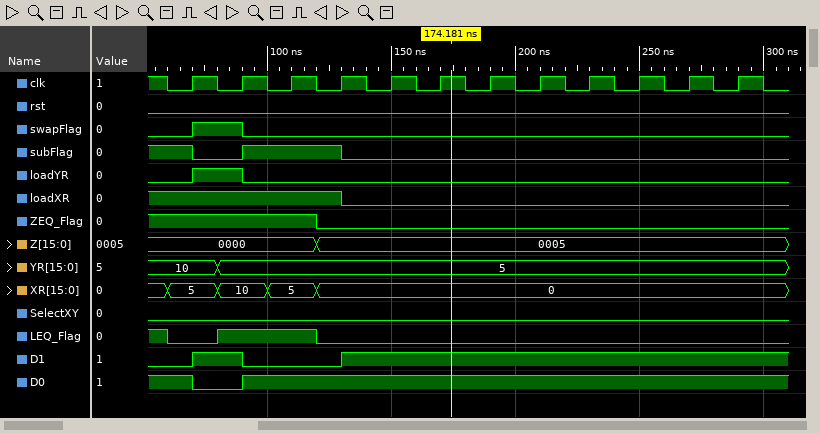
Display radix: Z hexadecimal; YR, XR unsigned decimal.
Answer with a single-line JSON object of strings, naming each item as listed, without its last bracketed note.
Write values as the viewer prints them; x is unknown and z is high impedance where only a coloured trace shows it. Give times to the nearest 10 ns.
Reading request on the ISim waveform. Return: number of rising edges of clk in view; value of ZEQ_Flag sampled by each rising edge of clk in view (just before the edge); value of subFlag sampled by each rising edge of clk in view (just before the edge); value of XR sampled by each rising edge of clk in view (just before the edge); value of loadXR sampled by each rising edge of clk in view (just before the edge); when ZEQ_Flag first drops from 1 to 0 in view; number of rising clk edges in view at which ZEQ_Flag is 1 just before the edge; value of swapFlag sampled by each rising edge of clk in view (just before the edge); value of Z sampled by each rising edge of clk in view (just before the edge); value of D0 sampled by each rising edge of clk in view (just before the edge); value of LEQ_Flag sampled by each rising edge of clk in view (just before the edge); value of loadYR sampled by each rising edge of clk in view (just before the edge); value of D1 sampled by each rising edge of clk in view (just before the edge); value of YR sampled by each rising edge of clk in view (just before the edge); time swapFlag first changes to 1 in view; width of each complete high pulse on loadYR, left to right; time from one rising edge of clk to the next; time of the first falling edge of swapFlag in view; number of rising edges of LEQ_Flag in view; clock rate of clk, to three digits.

{"number of rising edges of clk in view": "12", "value of ZEQ_Flag sampled by each rising edge of clk in view": "1 1 1 0 0 0 0 0 0 0 0 0", "value of subFlag sampled by each rising edge of clk in view": "1 0 1 1 0 0 0 0 0 0 0 0", "value of XR sampled by each rising edge of clk in view": "5, 10, 5, 0, 0, 0, 0, 0, 0, 0, 0, 0", "value of loadXR sampled by each rising edge of clk in view": "1 1 1 1 0 0 0 0 0 0 0 0", "when ZEQ_Flag first drops from 1 to 0 in view": "120 ns", "number of rising clk edges in view at which ZEQ_Flag is 1 just before the edge": "3", "value of swapFlag sampled by each rising edge of clk in view": "0 1 0 0 0 0 0 0 0 0 0 0", "value of Z sampled by each rising edge of clk in view": "0000, 0000, 0000, 0005, 0005, 0005, 0005, 0005, 0005, 0005, 0005, 0005", "value of D0 sampled by each rising edge of clk in view": "1 0 1 1 1 1 1 1 1 1 1 1", "value of LEQ_Flag sampled by each rising edge of clk in view": "0 1 1 0 0 0 0 0 0 0 0 0", "value of loadYR sampled by each rising edge of clk in view": "0 1 0 0 0 0 0 0 0 0 0 0", "value of D1 sampled by each rising edge of clk in view": "0 1 0 0 1 1 1 1 1 1 1 1", "value of YR sampled by each rising edge of clk in view": "10, 5, 5, 5, 5, 5, 5, 5, 5, 5, 5, 5", "time swapFlag first changes to 1 in view": "70 ns", "width of each complete high pulse on loadYR, left to right": "20 ns", "time from one rising edge of clk to the next": "20 ns", "time of the first falling edge of swapFlag in view": "90 ns", "number of rising edges of LEQ_Flag in view": "1", "clock rate of clk, to three digits": "50.0 MHz"}
